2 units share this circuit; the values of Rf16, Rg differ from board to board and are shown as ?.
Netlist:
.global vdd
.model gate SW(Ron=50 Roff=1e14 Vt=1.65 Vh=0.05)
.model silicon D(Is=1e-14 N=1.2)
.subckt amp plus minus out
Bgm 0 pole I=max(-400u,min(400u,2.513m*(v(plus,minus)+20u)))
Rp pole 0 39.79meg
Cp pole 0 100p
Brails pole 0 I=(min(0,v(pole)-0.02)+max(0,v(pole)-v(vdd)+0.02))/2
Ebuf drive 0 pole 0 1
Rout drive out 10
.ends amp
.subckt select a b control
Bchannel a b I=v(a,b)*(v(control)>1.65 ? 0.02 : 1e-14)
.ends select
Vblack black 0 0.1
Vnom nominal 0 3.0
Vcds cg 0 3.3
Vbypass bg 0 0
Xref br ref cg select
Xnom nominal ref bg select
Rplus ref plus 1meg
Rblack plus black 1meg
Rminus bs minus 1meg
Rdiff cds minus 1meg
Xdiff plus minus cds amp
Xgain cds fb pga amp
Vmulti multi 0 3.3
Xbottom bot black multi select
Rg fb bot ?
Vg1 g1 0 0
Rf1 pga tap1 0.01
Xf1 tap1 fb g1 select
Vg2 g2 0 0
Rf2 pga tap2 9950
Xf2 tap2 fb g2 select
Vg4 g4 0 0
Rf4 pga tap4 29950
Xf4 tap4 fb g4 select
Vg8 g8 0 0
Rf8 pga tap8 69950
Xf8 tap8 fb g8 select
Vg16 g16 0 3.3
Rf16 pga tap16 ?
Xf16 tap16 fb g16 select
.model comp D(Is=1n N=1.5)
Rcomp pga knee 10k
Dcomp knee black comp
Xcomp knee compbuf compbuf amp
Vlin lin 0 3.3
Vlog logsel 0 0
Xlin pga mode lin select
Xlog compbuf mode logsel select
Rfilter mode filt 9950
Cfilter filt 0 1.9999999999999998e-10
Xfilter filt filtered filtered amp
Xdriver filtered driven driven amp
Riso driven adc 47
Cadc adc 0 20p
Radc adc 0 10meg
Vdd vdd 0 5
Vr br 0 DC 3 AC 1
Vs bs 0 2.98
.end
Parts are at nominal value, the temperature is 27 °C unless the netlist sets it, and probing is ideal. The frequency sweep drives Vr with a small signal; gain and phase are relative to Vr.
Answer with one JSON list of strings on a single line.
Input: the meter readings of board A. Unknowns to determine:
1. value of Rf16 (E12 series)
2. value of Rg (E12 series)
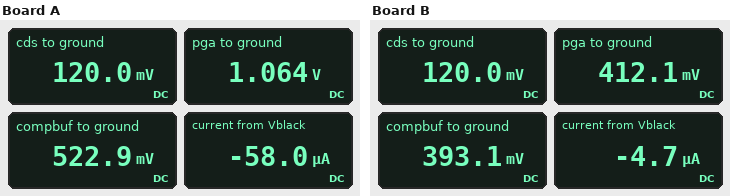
["390 kΩ", "8.2 kΩ"]
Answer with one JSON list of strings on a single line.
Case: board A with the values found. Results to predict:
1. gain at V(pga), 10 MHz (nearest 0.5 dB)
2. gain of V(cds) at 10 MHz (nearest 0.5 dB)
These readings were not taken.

["-22.0 dB", "-14.0 dB"]
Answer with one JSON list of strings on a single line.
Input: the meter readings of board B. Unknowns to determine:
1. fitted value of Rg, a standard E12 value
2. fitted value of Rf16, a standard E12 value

["15 kΩ", "220 kΩ"]
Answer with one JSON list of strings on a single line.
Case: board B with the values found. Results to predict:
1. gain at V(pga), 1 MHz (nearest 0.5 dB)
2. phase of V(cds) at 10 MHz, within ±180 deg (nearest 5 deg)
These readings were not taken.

["11.0 dB", "-80 deg"]
